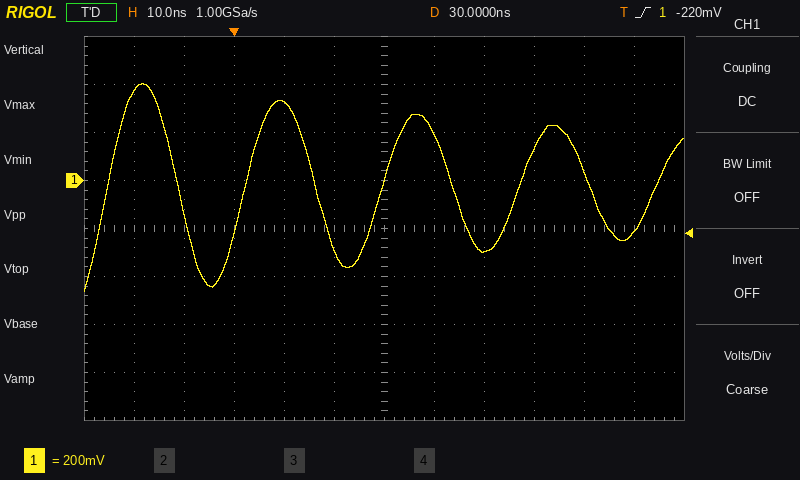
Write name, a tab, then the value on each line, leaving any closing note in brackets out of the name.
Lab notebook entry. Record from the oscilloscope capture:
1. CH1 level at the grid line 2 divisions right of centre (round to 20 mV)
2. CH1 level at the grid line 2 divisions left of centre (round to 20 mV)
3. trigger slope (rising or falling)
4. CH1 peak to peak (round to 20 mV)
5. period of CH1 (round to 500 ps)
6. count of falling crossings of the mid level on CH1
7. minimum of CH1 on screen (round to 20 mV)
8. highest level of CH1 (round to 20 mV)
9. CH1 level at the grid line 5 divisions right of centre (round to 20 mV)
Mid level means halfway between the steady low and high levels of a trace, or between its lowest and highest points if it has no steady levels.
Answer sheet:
CH1 level at the grid line 2 divisions right of centre	-300 mV
CH1 level at the grid line 2 divisions left of centre	320 mV
trigger slope	rising
CH1 peak to peak	860 mV
period of CH1	27.5 ns
count of falling crossings of the mid level on CH1	4
minimum of CH1 on screen	-460 mV
highest level of CH1	400 mV
CH1 level at the grid line 5 divisions right of centre	-220 mV
